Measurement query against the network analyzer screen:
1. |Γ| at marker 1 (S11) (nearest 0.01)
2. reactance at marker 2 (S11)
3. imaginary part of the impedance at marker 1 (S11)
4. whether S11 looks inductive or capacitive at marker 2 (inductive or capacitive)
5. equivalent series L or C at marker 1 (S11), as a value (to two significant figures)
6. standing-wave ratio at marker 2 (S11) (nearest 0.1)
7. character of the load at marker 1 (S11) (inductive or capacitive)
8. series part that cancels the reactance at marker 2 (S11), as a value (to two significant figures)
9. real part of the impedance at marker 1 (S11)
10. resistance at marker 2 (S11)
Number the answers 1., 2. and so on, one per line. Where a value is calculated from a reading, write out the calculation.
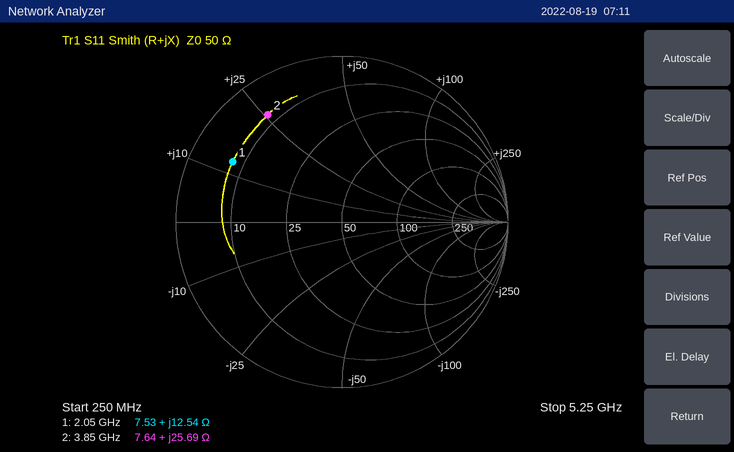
1. 0.75
2. +25.69 Ω
3. +12.54 Ω
4. inductive
5. L = 12.54 Ω/(2π × 2.05 GHz) ≈ 974 pH, so 970 pH to two significant figures
6. 8.3
7. inductive
8. C = 1/(2π × 3.85 GHz × 25.69 Ω) ≈ 1.6 pF
9. 7.53 Ω
10. 7.64 Ω
